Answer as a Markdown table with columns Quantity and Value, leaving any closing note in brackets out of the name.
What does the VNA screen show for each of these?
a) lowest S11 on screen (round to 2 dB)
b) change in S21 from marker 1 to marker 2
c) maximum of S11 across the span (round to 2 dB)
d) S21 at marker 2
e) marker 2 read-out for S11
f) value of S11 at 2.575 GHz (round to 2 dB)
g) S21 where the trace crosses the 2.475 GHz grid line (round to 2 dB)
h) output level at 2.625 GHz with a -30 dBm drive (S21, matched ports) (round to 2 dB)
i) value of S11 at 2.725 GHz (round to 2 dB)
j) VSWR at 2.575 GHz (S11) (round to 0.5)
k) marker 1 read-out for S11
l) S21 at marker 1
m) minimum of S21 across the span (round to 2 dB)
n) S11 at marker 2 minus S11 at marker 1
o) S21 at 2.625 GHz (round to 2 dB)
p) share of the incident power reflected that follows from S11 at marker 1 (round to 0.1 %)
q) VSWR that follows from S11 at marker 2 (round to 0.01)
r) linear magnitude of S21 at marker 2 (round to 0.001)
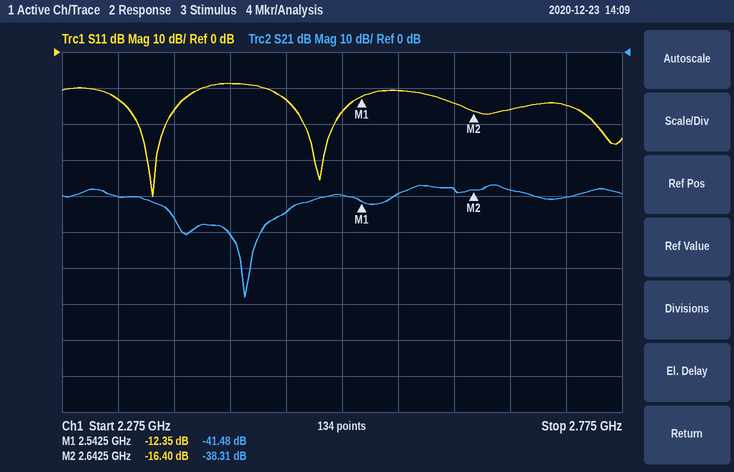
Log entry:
| Quantity | Value |
|---|---|
| lowest S11 on screen | -40 dB |
| change in S21 from marker 1 to marker 2 | 3.17 dB |
| maximum of S11 across the span | -8 dB |
| S21 at marker 2 | -38.31 dB |
| marker 2 read-out for S11 | -16.40 dB |
| value of S11 at 2.575 GHz | -10 dB |
| S21 where the trace crosses the 2.475 GHz grid line | -44 dB |
| output level at 2.625 GHz with a -30 dBm drive (S21, matched ports) | -68 dBm |
| value of S11 at 2.725 GHz | -14 dB |
| VSWR at 2.575 GHz (S11) | 2.0 |
| marker 1 read-out for S11 | -12.35 dB |
| S21 at marker 1 | -41.48 dB |
| minimum of S21 across the span | -68 dB |
| S11 at marker 2 minus S11 at marker 1 | -4.05 dB |
| S21 at 2.625 GHz | -38 dB |
| share of the incident power reflected that follows from S11 at marker 1 | 5.8 % |
| VSWR that follows from S11 at marker 2 | 1.36 |
| linear magnitude of S21 at marker 2 | 0.012 |
